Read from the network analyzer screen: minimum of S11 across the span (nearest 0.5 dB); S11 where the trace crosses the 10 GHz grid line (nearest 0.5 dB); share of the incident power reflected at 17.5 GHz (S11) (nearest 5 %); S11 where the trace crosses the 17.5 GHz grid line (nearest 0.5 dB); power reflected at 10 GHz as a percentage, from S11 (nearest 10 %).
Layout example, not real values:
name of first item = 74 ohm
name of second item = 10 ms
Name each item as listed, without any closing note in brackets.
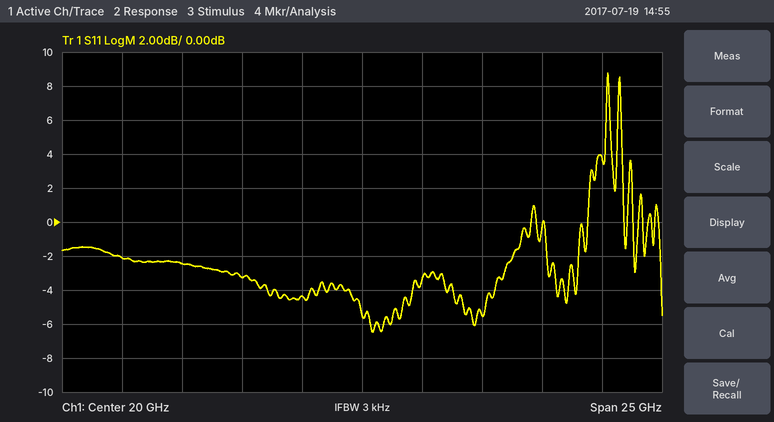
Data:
minimum of S11 across the span = -6.5 dB
S11 where the trace crosses the 10 GHz grid line = -2.0 dB
share of the incident power reflected at 17.5 GHz (S11) = 35 %
S11 where the trace crosses the 17.5 GHz grid line = -4.5 dB
power reflected at 10 GHz as a percentage, from S11 = 60 %
